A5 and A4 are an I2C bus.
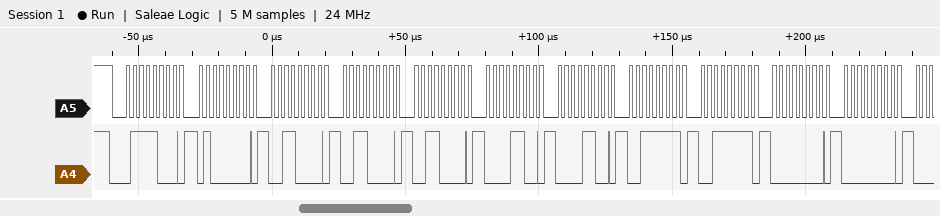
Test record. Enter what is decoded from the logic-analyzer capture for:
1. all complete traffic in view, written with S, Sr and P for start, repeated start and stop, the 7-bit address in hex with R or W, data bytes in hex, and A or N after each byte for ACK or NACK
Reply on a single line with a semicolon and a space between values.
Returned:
S 3CW A 40 A 30 A 30 A 30 A 0C A 0C A 3F A 3F A 00 A 00 A
